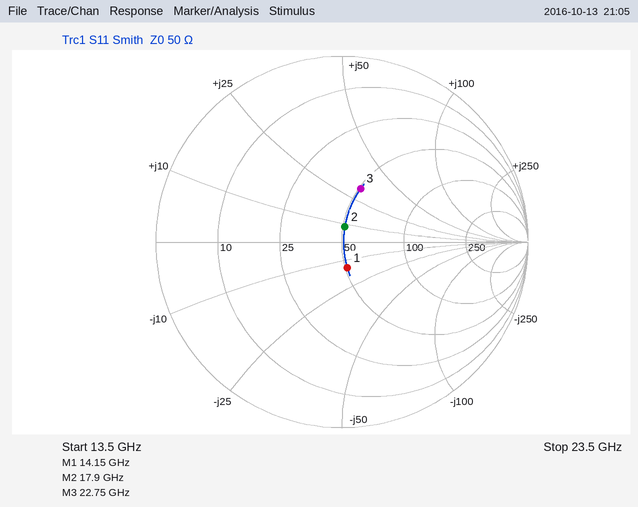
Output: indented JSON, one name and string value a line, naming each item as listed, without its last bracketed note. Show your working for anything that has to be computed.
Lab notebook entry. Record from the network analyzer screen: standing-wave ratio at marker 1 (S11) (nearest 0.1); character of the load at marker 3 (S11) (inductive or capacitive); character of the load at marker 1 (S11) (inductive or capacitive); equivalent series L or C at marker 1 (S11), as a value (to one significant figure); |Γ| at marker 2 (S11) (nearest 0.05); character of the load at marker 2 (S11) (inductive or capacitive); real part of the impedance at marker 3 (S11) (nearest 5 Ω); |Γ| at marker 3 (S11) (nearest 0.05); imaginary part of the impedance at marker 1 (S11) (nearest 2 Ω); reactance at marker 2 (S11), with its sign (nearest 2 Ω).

{
  "standing-wave ratio at marker 1 (S11)": "1.3",
  "character of the load at marker 3 (S11)": "inductive",
  "character of the load at marker 1 (S11)": "capacitive",
  "equivalent series L or C at marker 1 (S11), as a value": "C = 1/(2π × 14.15 GHz × 14 Ω) ≈ 803 fF, so 800 fF to one significant figure",
  "|Γ| at marker 2 (S11)": "0.10",
  "character of the load at marker 2 (S11)": "inductive",
  "real part of the impedance at marker 3 (S11)": "50 Ω",
  "|Γ| at marker 3 (S11)": "0.30",
  "imaginary part of the impedance at marker 1 (S11)": "-14 Ω",
  "reactance at marker 2 (S11), with its sign": "+8 Ω"
}
